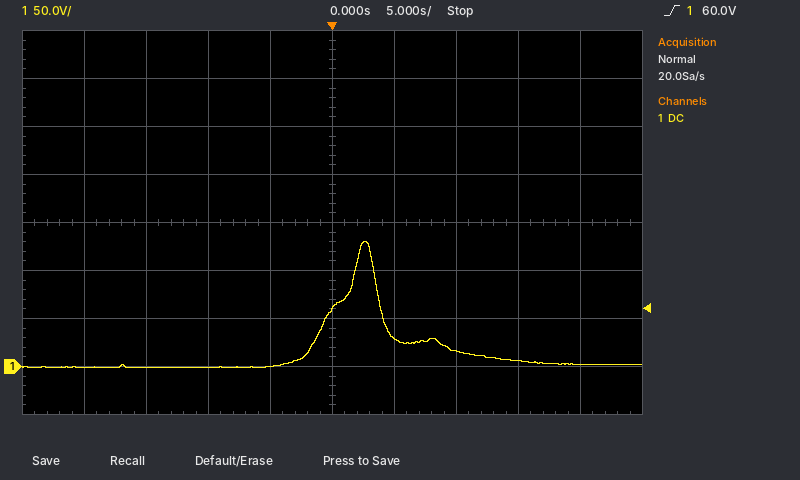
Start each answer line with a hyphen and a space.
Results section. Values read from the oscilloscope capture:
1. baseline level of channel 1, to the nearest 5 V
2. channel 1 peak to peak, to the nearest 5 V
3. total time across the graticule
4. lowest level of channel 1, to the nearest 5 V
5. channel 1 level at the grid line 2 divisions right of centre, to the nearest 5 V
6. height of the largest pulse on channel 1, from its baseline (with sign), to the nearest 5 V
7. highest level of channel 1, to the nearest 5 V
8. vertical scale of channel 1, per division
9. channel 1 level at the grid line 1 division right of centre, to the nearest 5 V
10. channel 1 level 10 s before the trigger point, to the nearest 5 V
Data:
- 0 V
- 130 V
- 50 s
- 0 V
- 15 V
- +130 V
- 130 V
- 50 V
- 30 V
- 0 V
